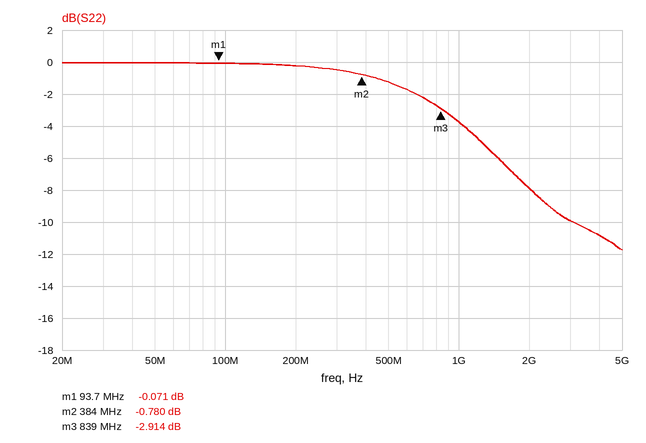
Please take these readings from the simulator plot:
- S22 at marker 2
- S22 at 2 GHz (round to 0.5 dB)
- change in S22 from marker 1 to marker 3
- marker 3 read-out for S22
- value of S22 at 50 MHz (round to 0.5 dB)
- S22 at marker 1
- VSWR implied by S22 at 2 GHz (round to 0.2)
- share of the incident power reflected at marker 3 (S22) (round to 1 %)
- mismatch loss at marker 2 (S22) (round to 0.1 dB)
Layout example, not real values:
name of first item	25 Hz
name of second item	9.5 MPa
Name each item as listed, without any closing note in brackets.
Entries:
S22 at marker 2	-0.780 dB
S22 at 2 GHz	-8.0 dB
change in S22 from marker 1 to marker 3	-2.843 dB
marker 3 read-out for S22	-2.914 dB
value of S22 at 50 MHz	0.0 dB
S22 at marker 1	-0.071 dB
VSWR implied by S22 at 2 GHz	2.4
share of the incident power reflected at marker 3 (S22)	51 %
mismatch loss at marker 2 (S22)	7.8 dB
